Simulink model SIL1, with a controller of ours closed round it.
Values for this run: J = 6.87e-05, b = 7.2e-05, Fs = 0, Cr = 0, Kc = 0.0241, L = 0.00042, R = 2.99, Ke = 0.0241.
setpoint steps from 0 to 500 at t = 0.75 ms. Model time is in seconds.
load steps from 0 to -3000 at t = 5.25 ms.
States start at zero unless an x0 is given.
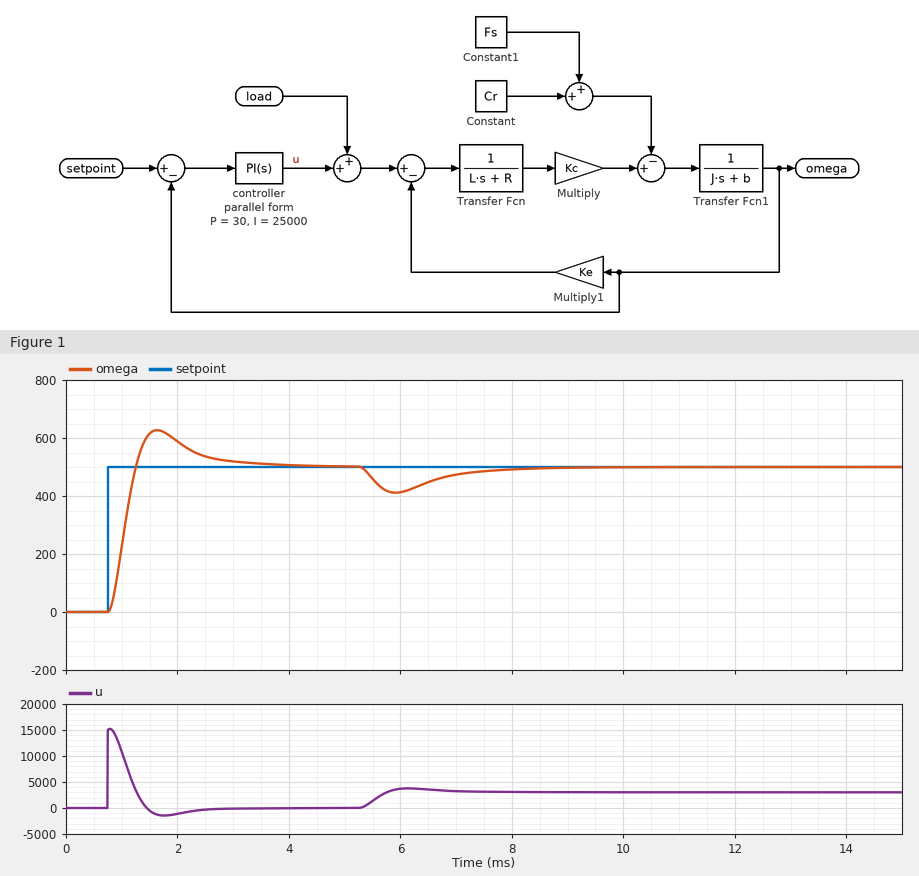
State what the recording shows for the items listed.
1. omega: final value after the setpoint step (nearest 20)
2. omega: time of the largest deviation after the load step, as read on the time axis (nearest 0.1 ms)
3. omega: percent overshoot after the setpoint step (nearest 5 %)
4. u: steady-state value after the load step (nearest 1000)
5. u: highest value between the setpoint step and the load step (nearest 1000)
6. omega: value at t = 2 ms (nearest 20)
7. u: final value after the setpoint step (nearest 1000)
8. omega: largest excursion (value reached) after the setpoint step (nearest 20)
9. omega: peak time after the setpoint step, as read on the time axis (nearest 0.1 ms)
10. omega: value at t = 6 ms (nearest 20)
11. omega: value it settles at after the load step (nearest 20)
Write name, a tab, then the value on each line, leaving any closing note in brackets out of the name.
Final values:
omega: final value after the setpoint step	500
omega: time of the largest deviation after the load step, as read on the time axis	5.9 ms
omega: percent overshoot after the setpoint step	25 %
u: steady-state value after the load step	3000
u: highest value between the setpoint step and the load step	15000
omega: value at t = 2 ms	580
u: final value after the setpoint step	0
omega: largest excursion (value reached) after the setpoint step	620
omega: peak time after the setpoint step, as read on the time axis	1.6 ms
omega: value at t = 6 ms	420
omega: value it settles at after the load step	500
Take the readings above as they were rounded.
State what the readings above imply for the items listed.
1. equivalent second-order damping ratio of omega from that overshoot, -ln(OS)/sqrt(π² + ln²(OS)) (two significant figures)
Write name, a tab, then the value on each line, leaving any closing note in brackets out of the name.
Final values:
equivalent second-order damping ratio of omega from that overshoot, -ln(OS)/sqrt(π² + ln²(OS))	0.40
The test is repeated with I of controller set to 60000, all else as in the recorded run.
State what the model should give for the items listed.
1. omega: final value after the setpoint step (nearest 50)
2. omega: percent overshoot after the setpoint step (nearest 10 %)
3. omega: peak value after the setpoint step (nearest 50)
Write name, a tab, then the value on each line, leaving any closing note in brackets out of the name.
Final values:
omega: final value after the setpoint step	500
omega: percent overshoot after the setpoint step	50 %
omega: peak value after the setpoint step	750
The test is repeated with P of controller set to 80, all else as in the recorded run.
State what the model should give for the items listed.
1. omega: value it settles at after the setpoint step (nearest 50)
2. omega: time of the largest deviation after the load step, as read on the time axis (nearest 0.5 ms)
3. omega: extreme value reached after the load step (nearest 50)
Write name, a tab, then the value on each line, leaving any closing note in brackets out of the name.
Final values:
omega: value it settles at after the setpoint step	500
omega: time of the largest deviation after the load step, as read on the time axis	5.5 ms
omega: extreme value reached after the load step	450
